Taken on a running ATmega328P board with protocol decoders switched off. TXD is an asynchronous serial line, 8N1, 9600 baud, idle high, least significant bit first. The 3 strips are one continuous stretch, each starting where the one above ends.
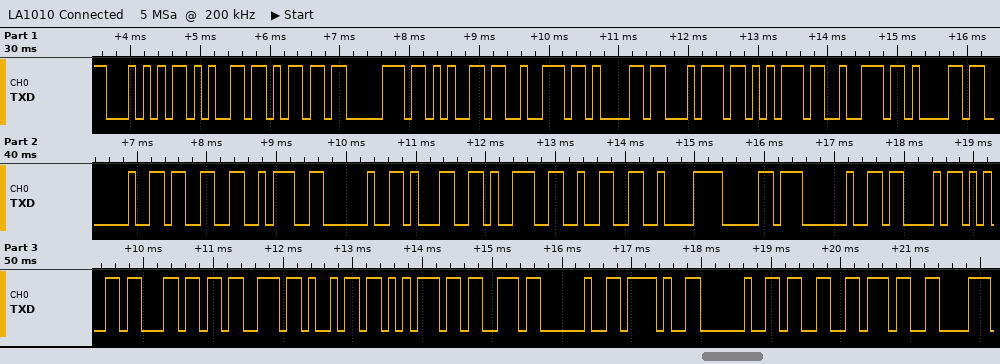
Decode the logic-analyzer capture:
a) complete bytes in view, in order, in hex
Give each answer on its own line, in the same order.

54 65 6D 70 65 72 61 74 75 72 61 20 33 3A 20 31 39 32 C2 B0 20 43 65 6C 73 69 75 73 20 2F 20 33 37
